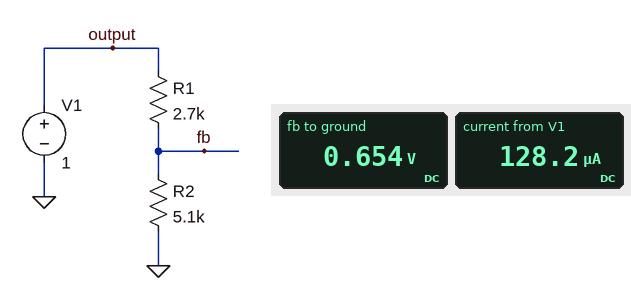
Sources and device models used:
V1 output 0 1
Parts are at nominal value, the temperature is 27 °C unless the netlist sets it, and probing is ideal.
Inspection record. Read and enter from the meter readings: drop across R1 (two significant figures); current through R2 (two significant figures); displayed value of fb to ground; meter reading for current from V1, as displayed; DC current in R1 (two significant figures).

350 mV
130 µA
0.654 V
128.2 µA
130 µA
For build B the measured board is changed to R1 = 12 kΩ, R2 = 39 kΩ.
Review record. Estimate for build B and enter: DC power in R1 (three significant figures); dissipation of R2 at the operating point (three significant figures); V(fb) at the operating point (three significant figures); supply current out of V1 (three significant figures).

4.61 µW
15.0 µW
765 mV
19.6 µA
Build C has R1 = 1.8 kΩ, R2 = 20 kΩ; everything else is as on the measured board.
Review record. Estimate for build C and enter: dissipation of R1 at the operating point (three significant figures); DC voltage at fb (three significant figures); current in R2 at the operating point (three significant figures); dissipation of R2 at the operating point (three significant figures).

3.79 µW
917 mV
45.9 µA
42.1 µW
